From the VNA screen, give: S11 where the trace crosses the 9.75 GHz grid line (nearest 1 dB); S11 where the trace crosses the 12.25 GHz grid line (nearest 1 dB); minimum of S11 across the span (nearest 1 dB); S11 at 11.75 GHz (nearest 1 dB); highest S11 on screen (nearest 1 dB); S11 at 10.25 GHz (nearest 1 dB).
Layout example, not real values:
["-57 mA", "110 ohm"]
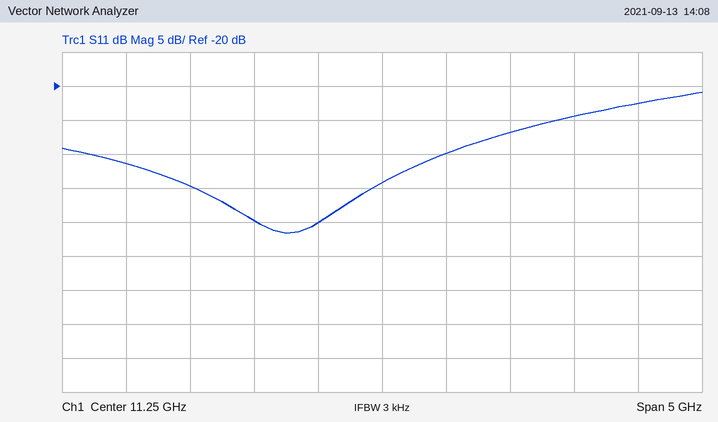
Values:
["-35 dB", "-27 dB", "-42 dB", "-30 dB", "-21 dB", "-40 dB"]
